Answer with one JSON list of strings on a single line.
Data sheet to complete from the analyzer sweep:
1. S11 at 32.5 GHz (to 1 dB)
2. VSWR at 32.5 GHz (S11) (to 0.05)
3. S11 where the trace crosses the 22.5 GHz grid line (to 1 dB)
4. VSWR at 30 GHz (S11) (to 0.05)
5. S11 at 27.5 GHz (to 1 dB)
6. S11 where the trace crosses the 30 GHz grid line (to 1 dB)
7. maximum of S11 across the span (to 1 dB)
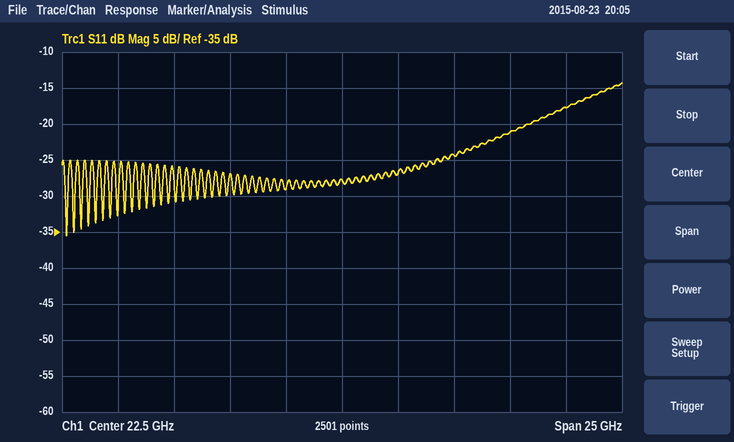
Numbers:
["-18 dB", "1.30", "-28 dB", "1.20", "-24 dB", "-21 dB", "-14 dB"]
